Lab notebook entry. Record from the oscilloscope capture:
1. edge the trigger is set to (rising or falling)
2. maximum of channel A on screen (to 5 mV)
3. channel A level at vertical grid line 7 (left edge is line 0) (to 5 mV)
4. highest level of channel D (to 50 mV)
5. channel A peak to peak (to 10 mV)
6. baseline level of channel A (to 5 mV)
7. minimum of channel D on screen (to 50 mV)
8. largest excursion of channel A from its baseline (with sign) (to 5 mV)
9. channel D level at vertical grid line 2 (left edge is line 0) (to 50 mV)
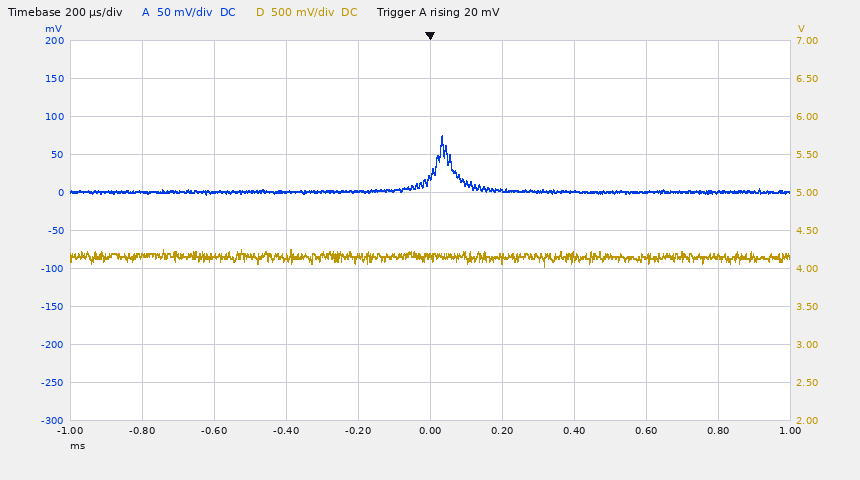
rising
75 mV
0 mV
4.25 V
80 mV
0 mV
4.05 V
+75 mV
4.15 V
